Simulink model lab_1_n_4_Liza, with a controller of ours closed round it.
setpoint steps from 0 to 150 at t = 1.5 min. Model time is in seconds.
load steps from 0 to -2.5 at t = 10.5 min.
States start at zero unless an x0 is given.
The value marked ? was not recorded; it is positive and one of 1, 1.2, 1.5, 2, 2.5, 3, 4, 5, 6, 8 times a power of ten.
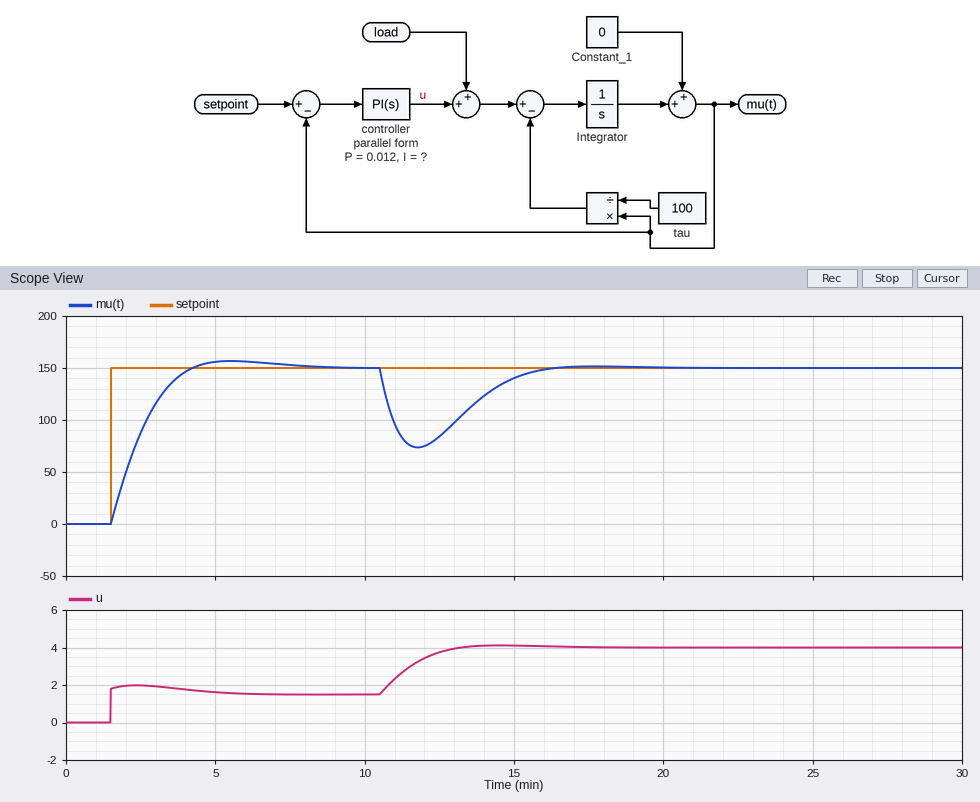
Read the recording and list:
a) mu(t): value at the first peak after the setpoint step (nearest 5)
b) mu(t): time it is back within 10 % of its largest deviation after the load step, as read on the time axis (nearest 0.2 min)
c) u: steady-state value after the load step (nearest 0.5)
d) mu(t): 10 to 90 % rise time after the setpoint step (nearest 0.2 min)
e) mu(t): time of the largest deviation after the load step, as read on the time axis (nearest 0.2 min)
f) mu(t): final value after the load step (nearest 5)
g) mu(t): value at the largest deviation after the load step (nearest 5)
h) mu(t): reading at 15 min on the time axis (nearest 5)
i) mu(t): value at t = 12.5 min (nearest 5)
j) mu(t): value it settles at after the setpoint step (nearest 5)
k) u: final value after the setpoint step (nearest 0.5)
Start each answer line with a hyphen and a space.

- 155
- 15.2 min
- 4.0
- 1.8 min
- 11.8 min
- 150
- 75
- 140
- 85
- 150
- 1.5
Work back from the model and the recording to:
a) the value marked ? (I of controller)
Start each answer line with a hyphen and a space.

- 0.0002
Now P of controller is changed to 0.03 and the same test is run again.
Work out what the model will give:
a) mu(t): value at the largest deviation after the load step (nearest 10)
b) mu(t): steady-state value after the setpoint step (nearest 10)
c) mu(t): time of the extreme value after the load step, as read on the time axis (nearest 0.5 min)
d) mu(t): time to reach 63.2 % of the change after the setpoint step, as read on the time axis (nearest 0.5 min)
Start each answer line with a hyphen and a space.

- 100
- 150
- 11.5 min
- 2.0 min
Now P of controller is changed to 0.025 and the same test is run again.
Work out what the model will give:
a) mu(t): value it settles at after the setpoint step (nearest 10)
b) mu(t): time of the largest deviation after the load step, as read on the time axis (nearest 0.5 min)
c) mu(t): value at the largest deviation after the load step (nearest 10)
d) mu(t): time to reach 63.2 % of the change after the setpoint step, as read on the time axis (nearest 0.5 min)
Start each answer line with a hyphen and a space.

- 150
- 11.5 min
- 90
- 2.0 min
